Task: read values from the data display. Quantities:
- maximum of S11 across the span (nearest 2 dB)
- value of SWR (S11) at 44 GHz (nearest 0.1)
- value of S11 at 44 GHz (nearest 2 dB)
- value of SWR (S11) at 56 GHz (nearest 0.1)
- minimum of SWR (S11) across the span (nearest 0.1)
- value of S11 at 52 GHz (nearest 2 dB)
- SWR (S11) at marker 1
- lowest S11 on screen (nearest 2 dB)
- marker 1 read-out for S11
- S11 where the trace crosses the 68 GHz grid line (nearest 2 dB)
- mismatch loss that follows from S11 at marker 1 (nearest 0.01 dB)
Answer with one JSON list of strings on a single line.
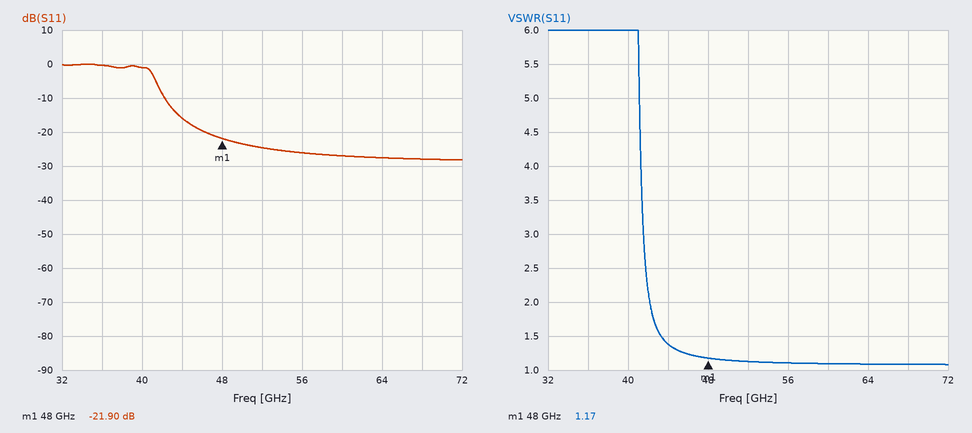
["0 dB", "1.4", "-16 dB", "1.1", "1.1", "-24 dB", "1.17", "-28 dB", "-21.90 dB", "-28 dB", "0.03 dB"]
